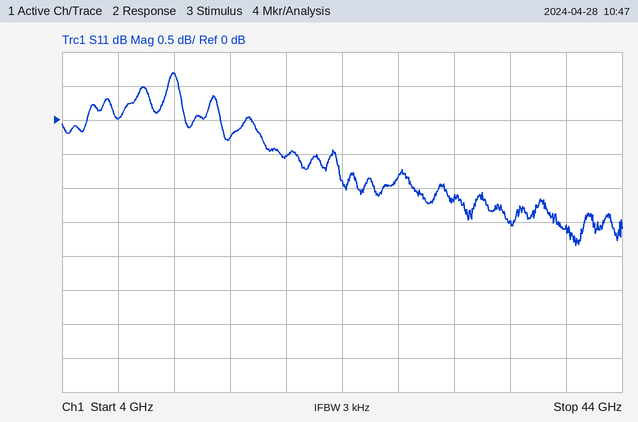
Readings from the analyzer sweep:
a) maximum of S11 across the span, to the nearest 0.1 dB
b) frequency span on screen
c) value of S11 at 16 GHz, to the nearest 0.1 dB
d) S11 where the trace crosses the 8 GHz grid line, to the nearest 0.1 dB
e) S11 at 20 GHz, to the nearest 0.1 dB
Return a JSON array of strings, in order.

["0.7 dB", "40 GHz", "-0.3 dB", "0.0 dB", "-0.5 dB"]
